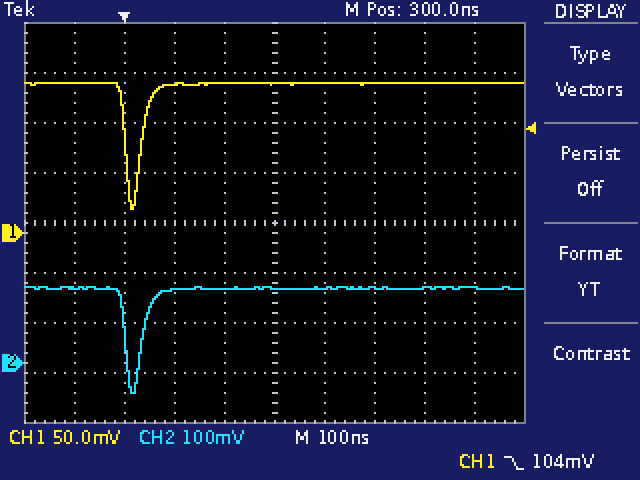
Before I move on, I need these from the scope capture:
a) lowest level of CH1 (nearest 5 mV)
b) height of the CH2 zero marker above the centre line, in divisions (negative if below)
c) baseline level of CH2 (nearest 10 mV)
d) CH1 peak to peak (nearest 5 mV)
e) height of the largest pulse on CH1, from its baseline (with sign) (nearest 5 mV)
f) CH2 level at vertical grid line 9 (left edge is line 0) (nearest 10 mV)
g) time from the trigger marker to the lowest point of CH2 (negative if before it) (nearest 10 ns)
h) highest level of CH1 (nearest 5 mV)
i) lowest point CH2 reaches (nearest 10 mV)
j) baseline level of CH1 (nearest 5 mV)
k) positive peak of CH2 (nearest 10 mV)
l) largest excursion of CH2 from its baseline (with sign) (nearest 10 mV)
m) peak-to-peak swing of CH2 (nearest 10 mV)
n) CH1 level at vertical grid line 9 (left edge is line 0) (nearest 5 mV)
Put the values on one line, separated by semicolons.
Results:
25 mV; -2.8 div; 150 mV; 125 mV; -125 mV; 150 mV; +20 ns; 150 mV; -60 mV; 150 mV; 150 mV; -210 mV; 210 mV; 150 mV
